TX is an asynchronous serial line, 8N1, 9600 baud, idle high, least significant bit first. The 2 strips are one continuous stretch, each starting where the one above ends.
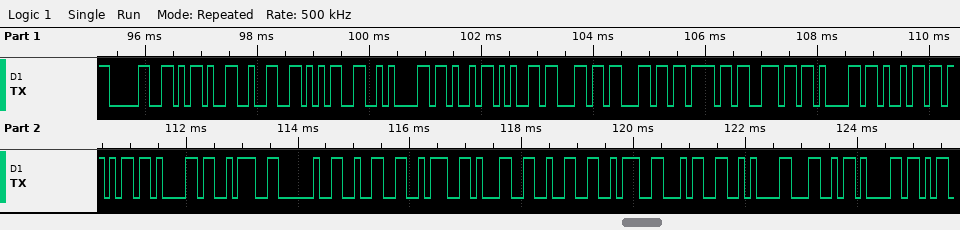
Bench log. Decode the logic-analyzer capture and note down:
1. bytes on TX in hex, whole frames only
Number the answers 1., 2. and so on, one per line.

1. 0x30 0x2D 0x32 0x35 0x0A 0x4B 0x65 0x6C 0x6C 0x6F 0x6E 0x61 0x69 0x6B 0x61 0x3A 0x20 0x32 0x3A 0x31 0x32 0x3A 0x34 0x0A 0x4C 0x61
